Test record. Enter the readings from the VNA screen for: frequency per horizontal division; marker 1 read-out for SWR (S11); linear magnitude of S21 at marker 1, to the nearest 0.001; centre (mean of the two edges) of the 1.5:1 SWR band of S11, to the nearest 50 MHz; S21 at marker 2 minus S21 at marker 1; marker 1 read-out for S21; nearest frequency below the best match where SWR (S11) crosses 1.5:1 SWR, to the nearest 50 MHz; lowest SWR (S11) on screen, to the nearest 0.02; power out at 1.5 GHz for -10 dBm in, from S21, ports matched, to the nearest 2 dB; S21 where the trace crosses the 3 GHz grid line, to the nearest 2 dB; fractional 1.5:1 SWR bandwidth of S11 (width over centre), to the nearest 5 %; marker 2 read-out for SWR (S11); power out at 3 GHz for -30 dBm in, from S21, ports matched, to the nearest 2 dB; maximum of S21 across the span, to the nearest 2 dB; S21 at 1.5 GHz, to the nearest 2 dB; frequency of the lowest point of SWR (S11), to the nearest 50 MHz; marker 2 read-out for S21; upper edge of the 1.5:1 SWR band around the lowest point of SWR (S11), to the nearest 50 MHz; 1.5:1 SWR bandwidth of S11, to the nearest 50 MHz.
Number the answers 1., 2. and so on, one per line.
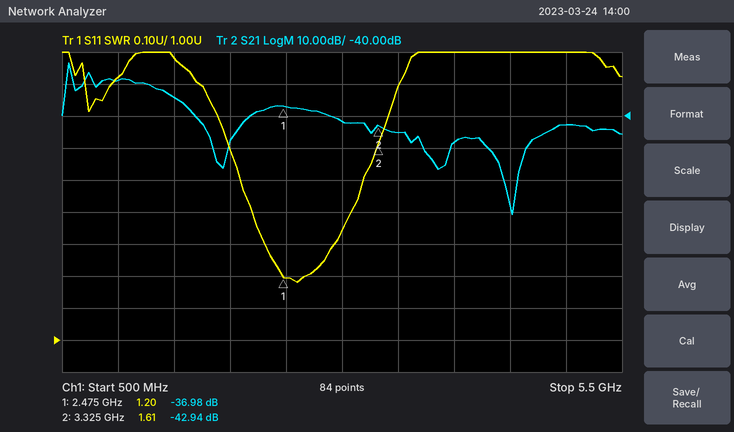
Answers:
1. 500 MHz
2. 1.20
3. 0.014
4. 2.65 GHz
5. -5.96 dB
6. -36.98 dB
7. 2.10 GHz
8. 1.18
9. -44 dBm
10. -42 dB
11. 40 %
12. 1.61
13. -72 dBm
14. -24 dB
15. -34 dB
16. 2.60 GHz
17. -42.94 dB
18. 3.20 GHz
19. 1.10 GHz
